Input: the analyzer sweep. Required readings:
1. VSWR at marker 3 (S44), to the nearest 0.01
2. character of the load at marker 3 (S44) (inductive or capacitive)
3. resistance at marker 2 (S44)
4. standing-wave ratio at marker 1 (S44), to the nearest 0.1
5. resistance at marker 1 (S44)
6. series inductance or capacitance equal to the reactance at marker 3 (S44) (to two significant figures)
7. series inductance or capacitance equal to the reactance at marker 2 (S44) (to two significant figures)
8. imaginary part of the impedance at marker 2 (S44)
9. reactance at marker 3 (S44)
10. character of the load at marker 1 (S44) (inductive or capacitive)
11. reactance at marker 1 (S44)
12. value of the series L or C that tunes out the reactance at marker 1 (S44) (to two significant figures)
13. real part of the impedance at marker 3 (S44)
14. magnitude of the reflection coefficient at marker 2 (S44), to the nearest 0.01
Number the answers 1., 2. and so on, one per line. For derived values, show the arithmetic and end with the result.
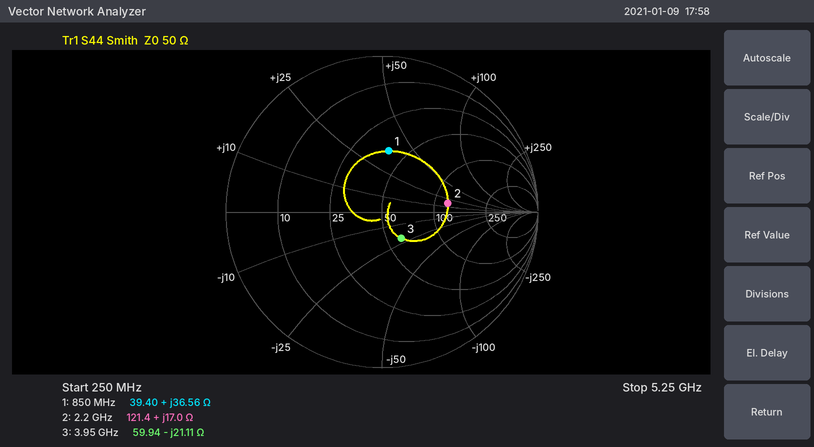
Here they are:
1. 1.53
2. capacitive
3. 121.4 Ω
4. 2.3
5. 39.40 Ω
6. C = 1/(2π × 3.95 GHz × 21.11 Ω) ≈ 1.9 pF
7. L = 17 Ω/(2π × 2.2 GHz) ≈ 1.2 nH
8. +17.0 Ω
9. -21.11 Ω
10. inductive
11. +36.56 Ω
12. C = 1/(2π × 850 MHz × 36.56 Ω) ≈ 5.1 pF
13. 59.94 Ω
14. 0.43
